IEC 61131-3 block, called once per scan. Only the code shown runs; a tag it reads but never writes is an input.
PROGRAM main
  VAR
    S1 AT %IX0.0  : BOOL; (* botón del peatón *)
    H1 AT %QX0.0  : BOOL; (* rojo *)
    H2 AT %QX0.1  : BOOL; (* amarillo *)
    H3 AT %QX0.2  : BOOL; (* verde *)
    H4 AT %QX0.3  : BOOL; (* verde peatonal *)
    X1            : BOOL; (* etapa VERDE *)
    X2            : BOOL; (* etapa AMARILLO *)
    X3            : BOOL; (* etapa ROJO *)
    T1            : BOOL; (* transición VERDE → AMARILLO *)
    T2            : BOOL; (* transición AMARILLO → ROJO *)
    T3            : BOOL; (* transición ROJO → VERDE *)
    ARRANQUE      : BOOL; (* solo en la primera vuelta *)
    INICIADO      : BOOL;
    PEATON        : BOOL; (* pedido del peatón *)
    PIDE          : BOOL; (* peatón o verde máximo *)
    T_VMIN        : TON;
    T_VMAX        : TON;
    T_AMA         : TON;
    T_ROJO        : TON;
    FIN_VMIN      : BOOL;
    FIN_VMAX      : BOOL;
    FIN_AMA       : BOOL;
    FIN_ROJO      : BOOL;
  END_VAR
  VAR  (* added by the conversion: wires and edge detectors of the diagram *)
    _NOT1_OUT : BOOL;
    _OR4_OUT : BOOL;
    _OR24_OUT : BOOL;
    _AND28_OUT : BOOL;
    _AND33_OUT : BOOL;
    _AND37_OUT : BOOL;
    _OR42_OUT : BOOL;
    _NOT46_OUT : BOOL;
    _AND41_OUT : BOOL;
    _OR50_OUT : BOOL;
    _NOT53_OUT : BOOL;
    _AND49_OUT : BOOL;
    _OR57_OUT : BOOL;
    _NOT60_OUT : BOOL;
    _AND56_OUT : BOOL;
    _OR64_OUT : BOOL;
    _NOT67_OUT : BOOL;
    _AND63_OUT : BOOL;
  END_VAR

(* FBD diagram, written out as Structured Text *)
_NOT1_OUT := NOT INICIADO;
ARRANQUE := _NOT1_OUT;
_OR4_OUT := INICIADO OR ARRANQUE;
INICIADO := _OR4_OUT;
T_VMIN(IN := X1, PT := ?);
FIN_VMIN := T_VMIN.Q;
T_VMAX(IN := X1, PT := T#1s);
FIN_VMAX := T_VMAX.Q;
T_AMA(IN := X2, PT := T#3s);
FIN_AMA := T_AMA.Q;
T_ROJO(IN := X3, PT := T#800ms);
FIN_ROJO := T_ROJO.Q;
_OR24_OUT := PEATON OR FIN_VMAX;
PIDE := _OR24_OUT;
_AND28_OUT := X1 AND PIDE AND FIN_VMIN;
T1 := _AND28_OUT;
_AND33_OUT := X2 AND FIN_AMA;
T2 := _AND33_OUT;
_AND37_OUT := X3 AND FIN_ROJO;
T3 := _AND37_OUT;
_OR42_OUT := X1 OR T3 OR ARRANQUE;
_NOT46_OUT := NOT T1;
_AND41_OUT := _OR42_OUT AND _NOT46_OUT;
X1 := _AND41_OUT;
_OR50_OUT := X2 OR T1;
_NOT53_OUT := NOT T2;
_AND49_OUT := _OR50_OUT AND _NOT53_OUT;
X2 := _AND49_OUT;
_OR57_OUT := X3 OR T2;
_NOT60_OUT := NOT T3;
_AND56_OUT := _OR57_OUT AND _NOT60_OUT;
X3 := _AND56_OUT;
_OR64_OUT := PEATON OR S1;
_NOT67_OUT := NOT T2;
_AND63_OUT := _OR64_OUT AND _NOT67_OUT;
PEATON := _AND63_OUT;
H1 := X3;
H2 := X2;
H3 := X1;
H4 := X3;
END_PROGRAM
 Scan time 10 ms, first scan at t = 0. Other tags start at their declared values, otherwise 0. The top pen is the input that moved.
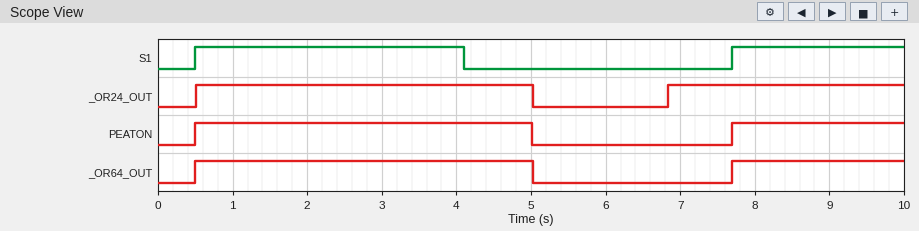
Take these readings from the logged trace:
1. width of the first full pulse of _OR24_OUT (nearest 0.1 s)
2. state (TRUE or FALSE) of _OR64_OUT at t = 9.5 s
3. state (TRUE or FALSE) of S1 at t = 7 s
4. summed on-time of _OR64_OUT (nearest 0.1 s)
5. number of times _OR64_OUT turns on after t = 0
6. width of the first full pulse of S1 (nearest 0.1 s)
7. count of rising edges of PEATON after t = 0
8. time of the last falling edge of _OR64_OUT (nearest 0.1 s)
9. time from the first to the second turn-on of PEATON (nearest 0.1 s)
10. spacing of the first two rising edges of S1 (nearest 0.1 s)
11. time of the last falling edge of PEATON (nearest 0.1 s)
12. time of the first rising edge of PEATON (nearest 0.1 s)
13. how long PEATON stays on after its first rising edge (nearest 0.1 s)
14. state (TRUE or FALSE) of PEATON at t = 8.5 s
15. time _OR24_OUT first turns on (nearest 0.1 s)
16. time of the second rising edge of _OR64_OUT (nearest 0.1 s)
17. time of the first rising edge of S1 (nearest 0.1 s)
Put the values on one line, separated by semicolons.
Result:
4.5 s; TRUE; FALSE; 6.8 s; 2; 3.6 s; 2; 5.0 s; 7.2 s; 7.2 s; 5.0 s; 0.5 s; 4.5 s; TRUE; 0.5 s; 7.7 s; 0.5 s
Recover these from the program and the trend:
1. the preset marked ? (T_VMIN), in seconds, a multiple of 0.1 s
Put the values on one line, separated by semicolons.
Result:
2.0 s
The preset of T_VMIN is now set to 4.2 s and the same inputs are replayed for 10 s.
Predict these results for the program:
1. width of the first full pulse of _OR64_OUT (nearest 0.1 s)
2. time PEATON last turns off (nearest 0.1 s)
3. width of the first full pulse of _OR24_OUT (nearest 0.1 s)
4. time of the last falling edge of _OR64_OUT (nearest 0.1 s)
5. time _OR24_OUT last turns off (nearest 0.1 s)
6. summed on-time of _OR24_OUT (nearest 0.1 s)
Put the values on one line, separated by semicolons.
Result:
6.7 s; 7.2 s; 6.7 s; 7.2 s; 7.2 s; 9.0 s
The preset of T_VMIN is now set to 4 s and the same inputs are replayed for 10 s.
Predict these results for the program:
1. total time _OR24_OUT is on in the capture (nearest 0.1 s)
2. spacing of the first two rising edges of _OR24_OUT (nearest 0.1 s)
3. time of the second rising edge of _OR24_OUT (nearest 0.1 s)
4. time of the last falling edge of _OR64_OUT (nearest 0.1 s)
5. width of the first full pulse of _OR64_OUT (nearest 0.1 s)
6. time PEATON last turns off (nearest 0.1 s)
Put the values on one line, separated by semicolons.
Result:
8.8 s; 7.2 s; 7.7 s; 7.0 s; 6.5 s; 7.0 s
